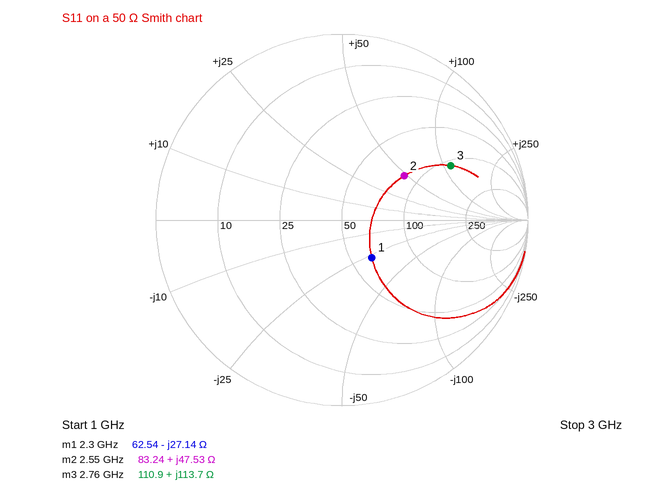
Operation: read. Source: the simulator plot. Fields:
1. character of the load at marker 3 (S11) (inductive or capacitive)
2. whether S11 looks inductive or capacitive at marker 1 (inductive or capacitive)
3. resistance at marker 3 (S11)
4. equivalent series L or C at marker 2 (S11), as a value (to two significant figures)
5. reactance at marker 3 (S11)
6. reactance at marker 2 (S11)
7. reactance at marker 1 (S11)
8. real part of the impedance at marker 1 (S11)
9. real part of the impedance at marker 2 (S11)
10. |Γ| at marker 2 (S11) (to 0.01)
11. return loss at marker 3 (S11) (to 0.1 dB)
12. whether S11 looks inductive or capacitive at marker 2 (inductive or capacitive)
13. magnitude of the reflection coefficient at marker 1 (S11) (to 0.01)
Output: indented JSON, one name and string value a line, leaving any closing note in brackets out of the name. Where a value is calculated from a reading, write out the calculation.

{
  "character of the load at marker 3 (S11)": "inductive",
  "whether S11 looks inductive or capacitive at marker 1": "capacitive",
  "resistance at marker 3": "110.9 Ω",
  "equivalent series L or C at marker 2 (S11), as a value": "L = 47.53 Ω/(2π × 2.55 GHz) ≈ 3.0 nH",
  "reactance at marker 3": "+113.7 Ω",
  "reactance at marker 2": "+47.53 Ω",
  "reactance at marker 1": "-27.14 Ω",
  "real part of the impedance at marker 1": "62.54 Ω",
  "real part of the impedance at marker 2": "83.24 Ω",
  "|Γ| at marker 2 (S11)": "0.41",
  "return loss at marker 3 (S11)": "3.7 dB",
  "whether S11 looks inductive or capacitive at marker 2": "inductive",
  "magnitude of the reflection coefficient at marker 1 (S11)": "0.26"
}
